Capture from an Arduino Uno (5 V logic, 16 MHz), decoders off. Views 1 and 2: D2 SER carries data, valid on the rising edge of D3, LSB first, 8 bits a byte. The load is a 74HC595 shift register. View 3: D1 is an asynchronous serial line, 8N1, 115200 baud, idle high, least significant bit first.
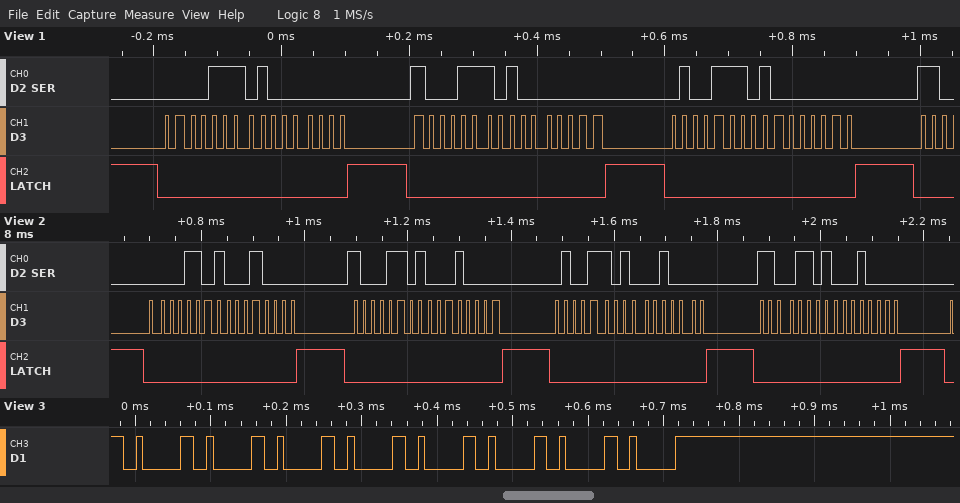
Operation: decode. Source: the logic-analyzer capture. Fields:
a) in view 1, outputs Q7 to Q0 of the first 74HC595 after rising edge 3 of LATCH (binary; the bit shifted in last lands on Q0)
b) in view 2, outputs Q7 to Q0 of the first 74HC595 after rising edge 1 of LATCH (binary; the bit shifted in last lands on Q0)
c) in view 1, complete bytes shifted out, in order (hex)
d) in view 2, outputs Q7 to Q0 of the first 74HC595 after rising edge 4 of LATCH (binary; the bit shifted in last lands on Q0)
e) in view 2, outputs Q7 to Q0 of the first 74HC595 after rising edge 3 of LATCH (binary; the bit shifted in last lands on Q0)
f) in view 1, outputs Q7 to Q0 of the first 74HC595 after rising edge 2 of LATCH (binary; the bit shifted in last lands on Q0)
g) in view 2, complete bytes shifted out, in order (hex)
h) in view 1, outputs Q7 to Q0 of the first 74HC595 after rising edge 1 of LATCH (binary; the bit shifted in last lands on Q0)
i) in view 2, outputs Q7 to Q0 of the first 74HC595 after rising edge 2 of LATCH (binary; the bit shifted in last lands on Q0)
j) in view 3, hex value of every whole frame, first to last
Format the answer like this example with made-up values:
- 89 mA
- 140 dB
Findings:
- 10000000
- 00010000
- 0x70 0x01 0x71 0x01 0x72 0x01
- 00010000
- 00010000
- 10000000
- B0 08 B1 08 B2 08 B3 08
- 10000000
- 00010000
- 02 02 02 02 02 02 02 02
